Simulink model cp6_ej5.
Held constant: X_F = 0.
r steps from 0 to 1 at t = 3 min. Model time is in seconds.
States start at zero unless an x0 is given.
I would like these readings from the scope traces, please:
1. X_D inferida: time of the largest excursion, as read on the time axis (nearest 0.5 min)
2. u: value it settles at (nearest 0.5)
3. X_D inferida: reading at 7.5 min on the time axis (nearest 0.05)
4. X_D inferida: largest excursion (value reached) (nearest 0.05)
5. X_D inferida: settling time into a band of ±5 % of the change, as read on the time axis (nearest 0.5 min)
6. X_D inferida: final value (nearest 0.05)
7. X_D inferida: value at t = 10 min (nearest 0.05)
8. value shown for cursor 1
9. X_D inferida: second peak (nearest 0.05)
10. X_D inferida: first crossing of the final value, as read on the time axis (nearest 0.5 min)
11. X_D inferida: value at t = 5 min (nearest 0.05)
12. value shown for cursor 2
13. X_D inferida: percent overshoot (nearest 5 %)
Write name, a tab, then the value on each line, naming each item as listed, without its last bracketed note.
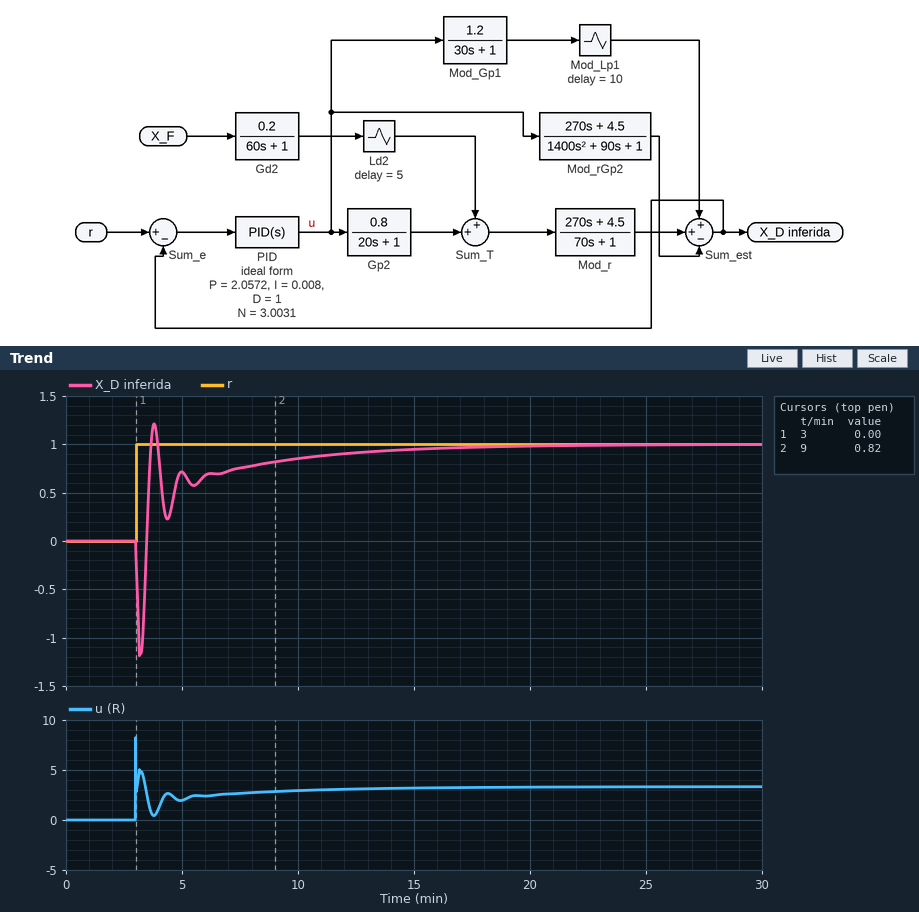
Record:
X_D inferida: time of the largest excursion, as read on the time axis	4.0 min
u: value it settles at	3.5
X_D inferida: reading at 7.5 min on the time axis	0.75
X_D inferida: largest excursion (value reached)	1.20
X_D inferida: settling time into a band of ±5 % of the change, as read on the time axis	15.0 min
X_D inferida: final value	1.00
X_D inferida: value at t = 10 min	0.85
value shown for cursor 1	0.00
X_D inferida: second peak	0.70
X_D inferida: first crossing of the final value, as read on the time axis	3.5 min
X_D inferida: value at t = 5 min	0.70
value shown for cursor 2	0.82
X_D inferida: percent overshoot	20 %
